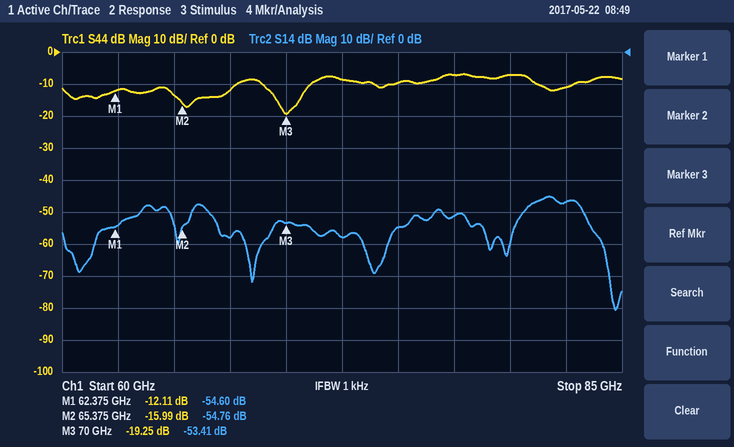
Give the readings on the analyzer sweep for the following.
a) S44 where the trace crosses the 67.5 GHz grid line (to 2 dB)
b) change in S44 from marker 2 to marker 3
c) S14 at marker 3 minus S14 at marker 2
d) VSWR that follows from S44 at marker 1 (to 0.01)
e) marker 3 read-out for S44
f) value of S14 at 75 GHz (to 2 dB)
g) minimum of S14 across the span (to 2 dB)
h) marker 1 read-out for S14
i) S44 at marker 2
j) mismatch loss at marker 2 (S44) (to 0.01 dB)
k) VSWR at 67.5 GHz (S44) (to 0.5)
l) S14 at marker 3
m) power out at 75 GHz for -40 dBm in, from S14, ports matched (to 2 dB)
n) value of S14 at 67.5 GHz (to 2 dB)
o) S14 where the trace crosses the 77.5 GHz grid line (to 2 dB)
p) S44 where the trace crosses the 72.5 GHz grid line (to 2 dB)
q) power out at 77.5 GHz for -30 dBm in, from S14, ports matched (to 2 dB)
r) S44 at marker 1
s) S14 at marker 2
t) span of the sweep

-12 dB
-3.26 dB
1.35 dB
1.66
-19.25 dB
-54 dB
-80 dB
-54.60 dB
-15.99 dB
0.11 dB
1.5
-53.41 dB
-94 dBm
-58 dB
-52 dB
-8 dB
-82 dBm
-12.11 dB
-54.76 dB
25 GHz
